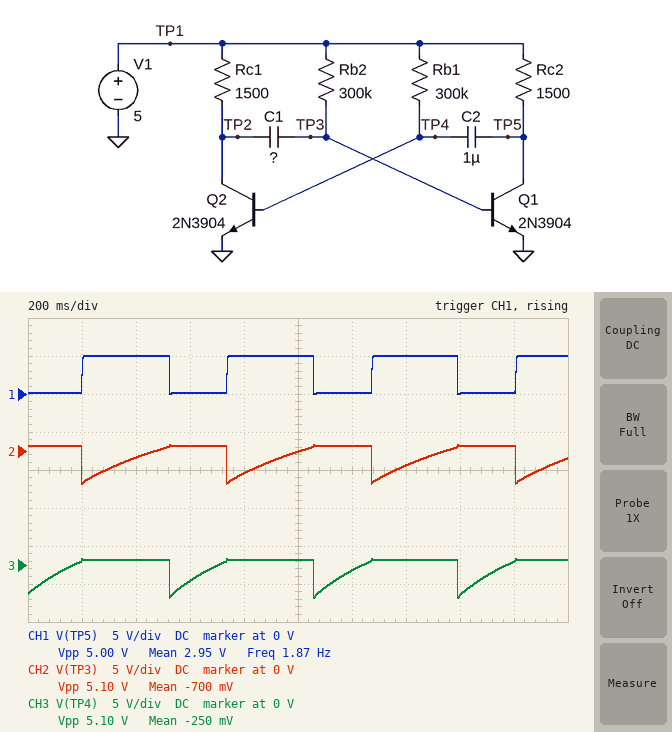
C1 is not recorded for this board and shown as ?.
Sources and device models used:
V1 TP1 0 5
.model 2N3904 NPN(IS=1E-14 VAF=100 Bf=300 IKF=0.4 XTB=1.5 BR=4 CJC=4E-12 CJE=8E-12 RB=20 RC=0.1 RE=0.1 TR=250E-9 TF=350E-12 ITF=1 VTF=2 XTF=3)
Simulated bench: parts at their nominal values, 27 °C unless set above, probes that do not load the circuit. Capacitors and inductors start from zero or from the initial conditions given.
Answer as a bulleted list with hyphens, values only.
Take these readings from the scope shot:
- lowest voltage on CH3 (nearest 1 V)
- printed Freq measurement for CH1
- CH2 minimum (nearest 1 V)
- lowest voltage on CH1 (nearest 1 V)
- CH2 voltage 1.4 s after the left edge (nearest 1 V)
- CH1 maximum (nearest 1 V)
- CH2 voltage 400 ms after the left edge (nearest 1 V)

- -4 V
- 1.87 Hz
- -4 V
- 0 V
- -2 V
- 5 V
- -1 V
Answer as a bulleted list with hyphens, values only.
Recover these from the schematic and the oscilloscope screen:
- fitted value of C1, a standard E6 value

- 1.5 µF
